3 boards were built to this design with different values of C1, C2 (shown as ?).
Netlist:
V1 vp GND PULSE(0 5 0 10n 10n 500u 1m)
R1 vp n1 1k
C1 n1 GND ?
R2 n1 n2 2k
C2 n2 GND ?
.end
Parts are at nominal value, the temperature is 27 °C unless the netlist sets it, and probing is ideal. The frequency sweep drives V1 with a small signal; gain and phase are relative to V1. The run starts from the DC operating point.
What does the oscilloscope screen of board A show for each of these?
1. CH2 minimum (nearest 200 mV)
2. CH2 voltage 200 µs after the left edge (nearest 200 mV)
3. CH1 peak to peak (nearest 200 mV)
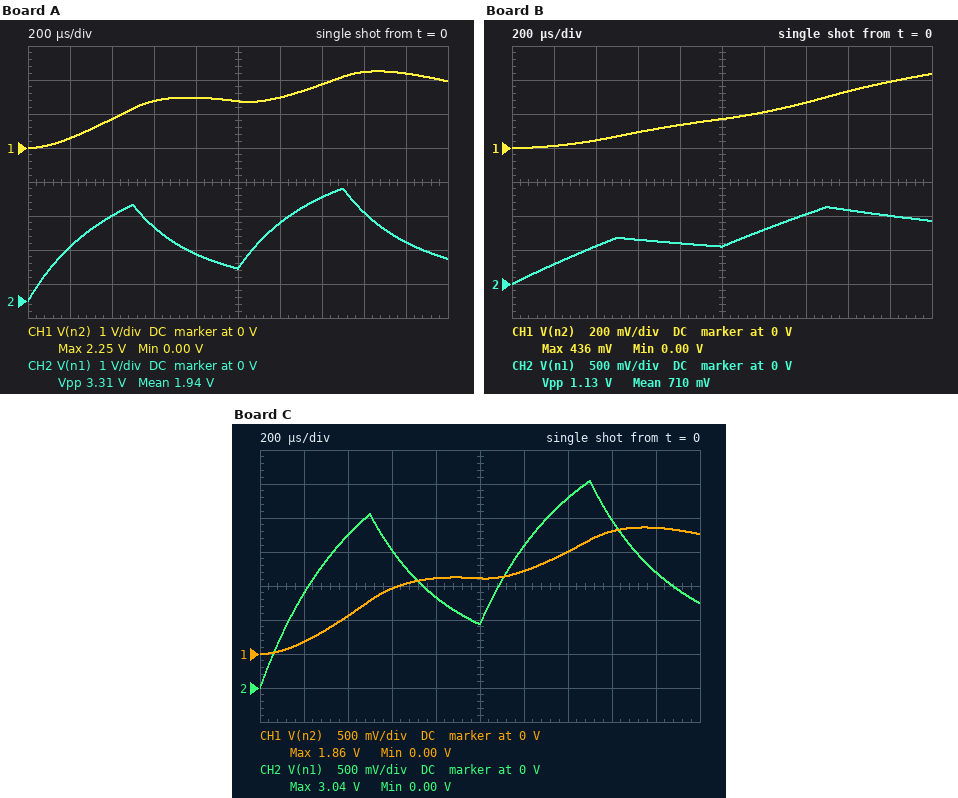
0 V
1.6 V
2.2 V
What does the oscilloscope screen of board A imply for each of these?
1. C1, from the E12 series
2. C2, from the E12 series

470 nF
270 nF
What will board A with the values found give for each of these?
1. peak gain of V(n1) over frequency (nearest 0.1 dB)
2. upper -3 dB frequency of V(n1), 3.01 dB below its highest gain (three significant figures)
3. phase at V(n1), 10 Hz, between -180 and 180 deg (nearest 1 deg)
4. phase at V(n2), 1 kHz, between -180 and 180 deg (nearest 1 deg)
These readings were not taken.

0 dB
198 Hz
-3 deg
-138 deg
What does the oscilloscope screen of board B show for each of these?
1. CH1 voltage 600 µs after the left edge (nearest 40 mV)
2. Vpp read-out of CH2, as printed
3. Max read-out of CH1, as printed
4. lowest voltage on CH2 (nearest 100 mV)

80 mV
1.13 V
436 mV
0 V
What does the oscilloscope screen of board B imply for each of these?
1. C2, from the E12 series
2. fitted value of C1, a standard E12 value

1.2 µF
3.3 µF
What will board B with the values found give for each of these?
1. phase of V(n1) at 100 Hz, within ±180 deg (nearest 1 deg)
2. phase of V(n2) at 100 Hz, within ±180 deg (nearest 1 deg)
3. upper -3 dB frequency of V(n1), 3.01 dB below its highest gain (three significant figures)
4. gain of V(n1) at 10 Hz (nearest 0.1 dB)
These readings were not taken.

-60 deg
-116 deg
33.2 Hz
-0.4 dB
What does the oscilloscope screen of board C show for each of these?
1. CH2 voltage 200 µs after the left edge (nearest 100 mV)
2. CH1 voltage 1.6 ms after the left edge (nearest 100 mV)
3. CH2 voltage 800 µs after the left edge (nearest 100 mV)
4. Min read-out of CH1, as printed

1.4 V
1.8 V
1.3 V
0.00 V
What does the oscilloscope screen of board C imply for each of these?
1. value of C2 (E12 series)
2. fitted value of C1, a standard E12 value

390 nF
560 nF
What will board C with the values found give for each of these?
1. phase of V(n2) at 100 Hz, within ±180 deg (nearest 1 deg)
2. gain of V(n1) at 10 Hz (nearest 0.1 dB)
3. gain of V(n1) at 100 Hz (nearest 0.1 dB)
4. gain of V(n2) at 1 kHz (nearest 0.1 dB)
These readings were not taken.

-53 deg
0 dB
-1.8 dB
-25.8 dB
